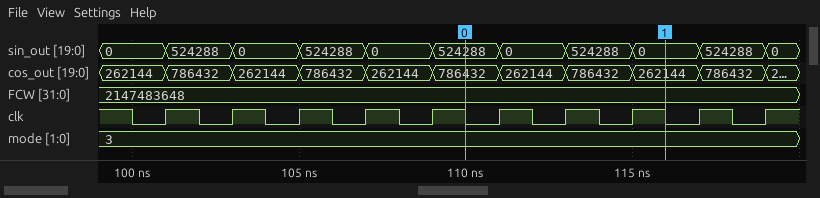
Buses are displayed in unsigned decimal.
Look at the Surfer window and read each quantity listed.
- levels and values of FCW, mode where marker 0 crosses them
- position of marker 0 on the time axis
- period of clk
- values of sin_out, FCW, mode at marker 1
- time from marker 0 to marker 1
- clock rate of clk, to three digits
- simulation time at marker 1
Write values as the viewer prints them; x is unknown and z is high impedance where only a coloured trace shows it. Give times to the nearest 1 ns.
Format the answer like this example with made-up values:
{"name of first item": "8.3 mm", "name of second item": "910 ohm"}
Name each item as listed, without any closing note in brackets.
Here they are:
{"levels and values of FCW, mode where marker 0 crosses them": "FCW=2147483648, mode=3", "position of marker 0 on the time axis": "110 ns", "period of clk": "2 ns", "values of sin_out, FCW, mode at marker 1": "sin_out=0, FCW=2147483648, mode=3", "time from marker 0 to marker 1": "6 ns", "clock rate of clk, to three digits": "500 MHz", "simulation time at marker 1": "116 ns"}
